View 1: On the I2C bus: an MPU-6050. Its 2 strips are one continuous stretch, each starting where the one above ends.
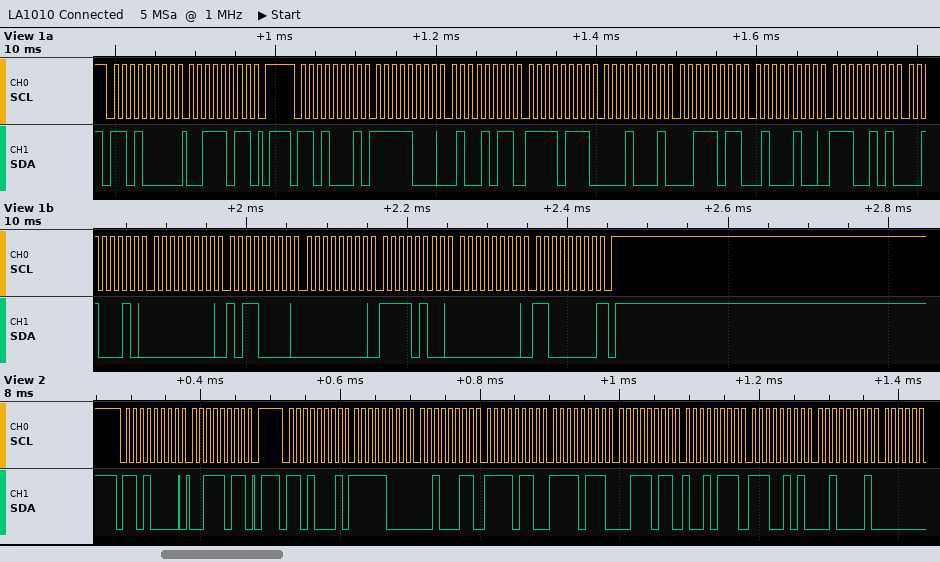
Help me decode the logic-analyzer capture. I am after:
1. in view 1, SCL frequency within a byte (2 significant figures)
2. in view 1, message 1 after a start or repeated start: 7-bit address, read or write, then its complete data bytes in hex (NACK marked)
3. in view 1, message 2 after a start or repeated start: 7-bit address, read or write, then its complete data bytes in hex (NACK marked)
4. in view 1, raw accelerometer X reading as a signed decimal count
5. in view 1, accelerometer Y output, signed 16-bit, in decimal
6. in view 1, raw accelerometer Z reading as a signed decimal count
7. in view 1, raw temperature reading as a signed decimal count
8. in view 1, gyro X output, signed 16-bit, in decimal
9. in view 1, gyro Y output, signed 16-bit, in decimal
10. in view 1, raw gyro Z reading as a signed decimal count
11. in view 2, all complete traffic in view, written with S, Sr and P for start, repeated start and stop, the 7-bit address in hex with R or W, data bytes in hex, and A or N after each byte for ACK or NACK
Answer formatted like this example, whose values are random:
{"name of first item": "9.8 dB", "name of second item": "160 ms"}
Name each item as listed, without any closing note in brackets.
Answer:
{"in view 1, SCL frequency within a byte": "100 kHz", "in view 1, message 1 after a start or repeated start: 7-bit address, read or write, then its complete data bytes in hex": "0x68 write: 3B", "in view 1, message 2 after a start or repeated start: 7-bit address, read or write, then its complete data bytes in hex": "0x68 read: F8 4B F7 11 3B 44 E5 22 00 B0 00 F4 00 C0 NACK", "in view 1, raw accelerometer X reading as a signed decimal count": "-1973", "in view 1, accelerometer Y output, signed 16-bit, in decimal": "-2287", "in view 1, raw accelerometer Z reading as a signed decimal count": "15172", "in view 1, raw temperature reading as a signed decimal count": "-6878", "in view 1, gyro X output, signed 16-bit, in decimal": "176", "in view 1, gyro Y output, signed 16-bit, in decimal": "244", "in view 1, raw gyro Z reading as a signed decimal count": "192", "in view 2, all complete traffic in view, written with S, Sr and P for start, repeated start and stop, the 7-bit address in hex with R or W, data bytes in hex, and A or N after each byte for ACK or NACK": "S 68W A 3B A P S 68R A F8 A 23 A F6 A F7 A 3B A 97 A E5 A 21 A"}
